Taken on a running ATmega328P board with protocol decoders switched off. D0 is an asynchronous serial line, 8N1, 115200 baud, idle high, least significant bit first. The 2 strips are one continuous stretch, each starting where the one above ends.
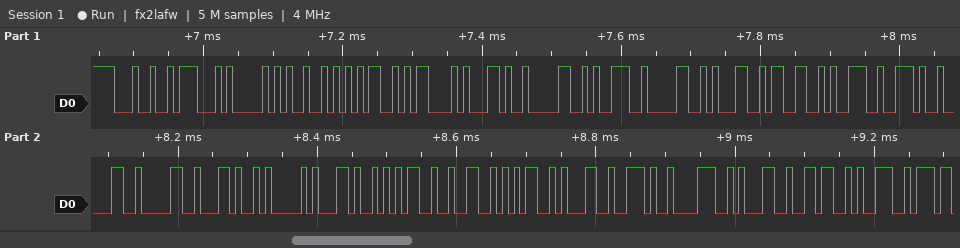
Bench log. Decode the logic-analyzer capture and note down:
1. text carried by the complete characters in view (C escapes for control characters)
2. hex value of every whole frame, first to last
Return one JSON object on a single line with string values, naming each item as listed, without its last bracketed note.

{"text carried by the complete characters in view": "\"$GPRMC,090139.00,A,5251.8169\"", "hex value of every whole frame, first to last": "24 47 50 52 4D 43 2C 30 39 30 31 33 39 2E 30 30 2C 41 2C 35 32 35 31 2E 38 31 36 39"}
